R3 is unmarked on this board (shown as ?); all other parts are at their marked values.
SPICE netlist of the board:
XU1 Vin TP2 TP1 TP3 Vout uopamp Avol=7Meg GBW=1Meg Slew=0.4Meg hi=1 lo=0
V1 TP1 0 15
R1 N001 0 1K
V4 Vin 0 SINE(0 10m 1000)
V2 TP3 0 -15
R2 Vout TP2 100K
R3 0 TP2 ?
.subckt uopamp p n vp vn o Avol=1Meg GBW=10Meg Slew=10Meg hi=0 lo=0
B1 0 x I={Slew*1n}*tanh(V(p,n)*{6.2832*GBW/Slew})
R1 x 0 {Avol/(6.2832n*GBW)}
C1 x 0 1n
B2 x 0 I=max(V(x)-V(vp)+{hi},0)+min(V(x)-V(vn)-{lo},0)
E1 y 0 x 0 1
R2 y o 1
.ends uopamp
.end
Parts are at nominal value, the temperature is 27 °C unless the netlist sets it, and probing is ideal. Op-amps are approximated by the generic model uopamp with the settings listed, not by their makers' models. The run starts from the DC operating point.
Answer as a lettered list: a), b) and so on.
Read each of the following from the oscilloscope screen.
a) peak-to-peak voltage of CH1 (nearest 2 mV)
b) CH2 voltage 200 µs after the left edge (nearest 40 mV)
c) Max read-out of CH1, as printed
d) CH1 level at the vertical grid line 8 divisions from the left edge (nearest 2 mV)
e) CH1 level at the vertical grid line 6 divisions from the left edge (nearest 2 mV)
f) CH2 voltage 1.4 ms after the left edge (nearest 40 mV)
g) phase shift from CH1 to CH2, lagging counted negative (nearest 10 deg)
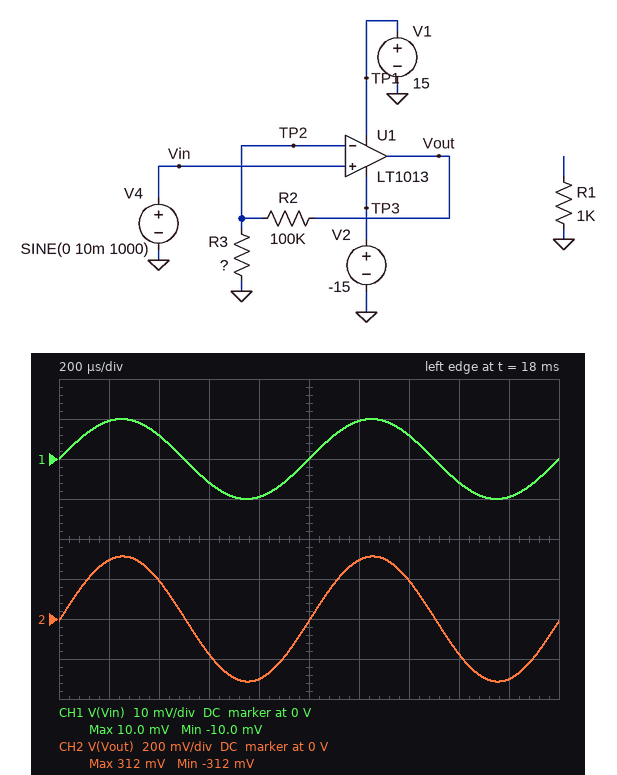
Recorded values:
a) 20 mV
b) 280 mV
c) 10.0 mV
d) -6 mV
e) 10 mV
f) 200 mV
g) 0 deg
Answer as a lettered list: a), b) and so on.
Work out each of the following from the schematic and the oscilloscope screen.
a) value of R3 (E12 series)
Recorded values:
a) 3.3 kΩ
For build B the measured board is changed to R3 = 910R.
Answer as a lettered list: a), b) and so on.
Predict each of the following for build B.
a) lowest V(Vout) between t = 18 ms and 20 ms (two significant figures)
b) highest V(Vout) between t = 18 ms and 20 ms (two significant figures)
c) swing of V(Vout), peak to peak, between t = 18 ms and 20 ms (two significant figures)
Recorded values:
a) -1.1 V
b) 1.1 V
c) 2.2 V
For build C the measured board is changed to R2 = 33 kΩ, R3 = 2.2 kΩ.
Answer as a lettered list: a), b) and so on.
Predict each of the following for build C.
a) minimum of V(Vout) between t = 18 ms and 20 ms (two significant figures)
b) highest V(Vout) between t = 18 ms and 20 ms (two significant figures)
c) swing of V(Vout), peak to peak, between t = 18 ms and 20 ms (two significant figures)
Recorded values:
a) -160 mV
b) 160 mV
c) 320 mV
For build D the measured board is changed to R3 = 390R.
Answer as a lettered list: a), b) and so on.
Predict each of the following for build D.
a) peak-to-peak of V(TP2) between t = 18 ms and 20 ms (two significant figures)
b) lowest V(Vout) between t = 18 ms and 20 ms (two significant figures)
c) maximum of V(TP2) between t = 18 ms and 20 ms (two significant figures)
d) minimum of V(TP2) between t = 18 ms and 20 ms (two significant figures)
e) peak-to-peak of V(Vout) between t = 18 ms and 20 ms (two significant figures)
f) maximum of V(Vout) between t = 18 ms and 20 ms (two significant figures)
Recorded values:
a) 19 mV
b) -2.5 V
c) 9.7 mV
d) -9.7 mV
e) 5.0 V
f) 2.5 V
